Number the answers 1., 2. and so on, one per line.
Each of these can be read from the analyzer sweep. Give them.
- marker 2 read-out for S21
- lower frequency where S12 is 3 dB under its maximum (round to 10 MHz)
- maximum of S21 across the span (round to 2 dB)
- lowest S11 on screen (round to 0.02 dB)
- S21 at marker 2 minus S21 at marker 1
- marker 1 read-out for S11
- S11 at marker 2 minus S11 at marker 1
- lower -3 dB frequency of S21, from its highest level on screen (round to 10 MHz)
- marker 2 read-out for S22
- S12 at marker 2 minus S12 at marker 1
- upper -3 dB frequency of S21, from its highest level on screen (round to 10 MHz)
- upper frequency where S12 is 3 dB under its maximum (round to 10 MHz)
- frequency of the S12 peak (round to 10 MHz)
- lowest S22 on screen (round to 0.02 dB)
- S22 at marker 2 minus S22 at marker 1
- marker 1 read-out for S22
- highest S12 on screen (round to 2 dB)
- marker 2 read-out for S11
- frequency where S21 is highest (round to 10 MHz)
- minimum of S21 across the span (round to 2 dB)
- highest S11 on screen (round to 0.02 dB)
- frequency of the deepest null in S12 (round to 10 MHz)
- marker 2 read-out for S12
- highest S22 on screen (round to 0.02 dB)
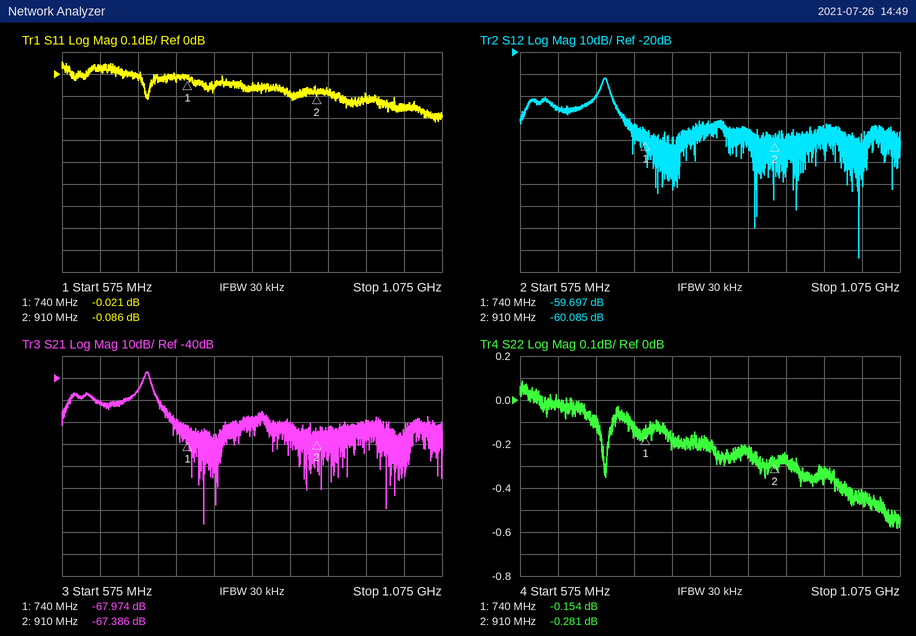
1. -67.386 dB
2. 680 MHz
3. -38 dB
4. -0.22 dB
5. 0.588 dB
6. -0.021 dB
7. -0.065 dB
8. 680 MHz
9. -0.281 dB
10. -0.388 dB
11. 690 MHz
12. 690 MHz
13. 690 MHz
14. -0.58 dB
15. -0.127 dB
16. -0.154 dB
17. -32 dB
18. -0.086 dB
19. 690 MHz
20. -106 dB
21. 0.06 dB
22. 1.02 GHz
23. -60.085 dB
24. 0.08 dB
